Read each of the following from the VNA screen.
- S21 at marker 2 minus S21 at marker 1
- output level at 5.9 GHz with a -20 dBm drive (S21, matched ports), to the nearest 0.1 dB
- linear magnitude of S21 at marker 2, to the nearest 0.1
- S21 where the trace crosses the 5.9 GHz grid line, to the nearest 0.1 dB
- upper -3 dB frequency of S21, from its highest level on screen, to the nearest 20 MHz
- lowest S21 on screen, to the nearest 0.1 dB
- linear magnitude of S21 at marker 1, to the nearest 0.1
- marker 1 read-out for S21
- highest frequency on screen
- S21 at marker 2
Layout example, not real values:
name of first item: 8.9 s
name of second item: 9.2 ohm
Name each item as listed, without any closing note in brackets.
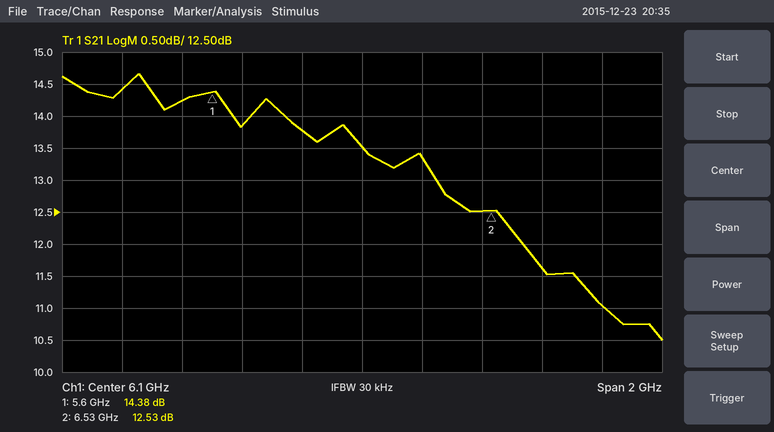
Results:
S21 at marker 2 minus S21 at marker 1: -1.85 dB
output level at 5.9 GHz with a -20 dBm drive (S21, matched ports), to the nearest 0.1 dB: -6.2 dBm
linear magnitude of S21 at marker 2, to the nearest 0.1: 4.2
S21 where the trace crosses the 5.9 GHz grid line, to the nearest 0.1 dB: 13.8 dB
upper -3 dB frequency of S21, from its highest level on screen, to the nearest 20 MHz: 6.70 GHz
lowest S21 on screen, to the nearest 0.1 dB: 10.5 dB
linear magnitude of S21 at marker 1, to the nearest 0.1: 5.2
marker 1 read-out for S21: 14.38 dB
highest frequency on screen: 7.1 GHz
S21 at marker 2: 12.53 dB
